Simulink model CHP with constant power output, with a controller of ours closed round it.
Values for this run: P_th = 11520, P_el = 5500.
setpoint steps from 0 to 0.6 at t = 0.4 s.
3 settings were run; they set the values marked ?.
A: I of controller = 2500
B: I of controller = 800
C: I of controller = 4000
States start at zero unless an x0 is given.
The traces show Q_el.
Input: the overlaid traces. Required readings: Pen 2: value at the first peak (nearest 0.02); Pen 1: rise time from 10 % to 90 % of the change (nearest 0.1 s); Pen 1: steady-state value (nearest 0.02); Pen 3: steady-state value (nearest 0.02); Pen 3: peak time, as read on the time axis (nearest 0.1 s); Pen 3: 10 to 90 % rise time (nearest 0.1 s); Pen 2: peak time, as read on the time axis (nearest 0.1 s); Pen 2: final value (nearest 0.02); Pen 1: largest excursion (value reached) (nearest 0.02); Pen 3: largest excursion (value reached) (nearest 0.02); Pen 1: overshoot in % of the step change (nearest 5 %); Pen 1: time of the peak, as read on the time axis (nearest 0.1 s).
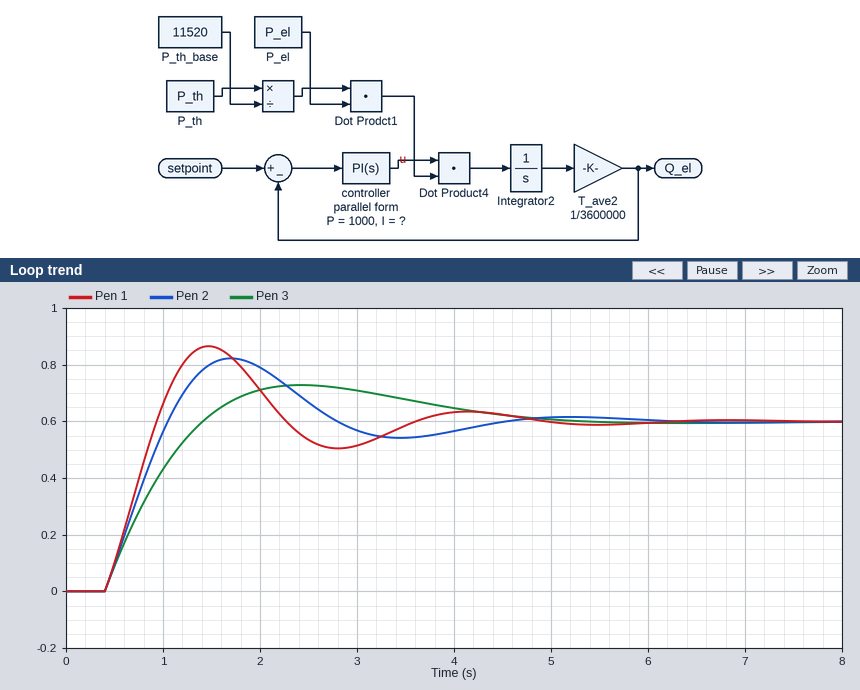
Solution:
0.82
0.4 s
0.60
0.60
2.4 s
0.8 s
1.7 s
0.60
0.86
0.72
45 %
1.5 s
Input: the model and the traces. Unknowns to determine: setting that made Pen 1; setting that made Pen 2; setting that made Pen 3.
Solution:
C
A
B
